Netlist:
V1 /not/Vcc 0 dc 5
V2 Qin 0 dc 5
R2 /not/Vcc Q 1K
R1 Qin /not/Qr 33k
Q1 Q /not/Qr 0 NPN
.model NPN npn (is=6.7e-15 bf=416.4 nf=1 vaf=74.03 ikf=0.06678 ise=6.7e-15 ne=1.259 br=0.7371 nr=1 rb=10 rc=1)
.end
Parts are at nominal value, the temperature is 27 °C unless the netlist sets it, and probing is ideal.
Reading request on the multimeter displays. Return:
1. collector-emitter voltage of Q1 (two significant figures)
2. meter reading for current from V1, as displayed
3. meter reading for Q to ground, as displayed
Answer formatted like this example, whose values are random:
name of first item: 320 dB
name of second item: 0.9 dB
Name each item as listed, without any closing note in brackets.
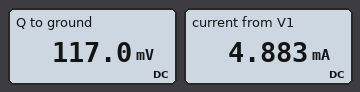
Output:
collector-emitter voltage of Q1: 120 mV
meter reading for current from V1, as displayed: 4.883 mA
meter reading for Q to ground, as displayed: 117.0 mV
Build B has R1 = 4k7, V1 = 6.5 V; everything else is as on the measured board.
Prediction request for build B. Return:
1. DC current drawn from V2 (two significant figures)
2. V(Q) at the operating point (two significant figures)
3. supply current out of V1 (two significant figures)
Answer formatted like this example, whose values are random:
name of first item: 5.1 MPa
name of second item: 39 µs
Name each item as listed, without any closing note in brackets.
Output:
DC current drawn from V2: 910 µA
V(Q) at the operating point: 75 mV
supply current out of V1: 6.4 mA
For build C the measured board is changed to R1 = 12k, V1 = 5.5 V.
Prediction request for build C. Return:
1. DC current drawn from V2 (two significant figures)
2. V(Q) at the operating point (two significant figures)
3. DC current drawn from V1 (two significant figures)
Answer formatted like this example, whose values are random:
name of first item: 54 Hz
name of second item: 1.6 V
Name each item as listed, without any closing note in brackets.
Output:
DC current drawn from V2: 360 µA
V(Q) at the operating point: 91 mV
DC current drawn from V1: 5.4 mA
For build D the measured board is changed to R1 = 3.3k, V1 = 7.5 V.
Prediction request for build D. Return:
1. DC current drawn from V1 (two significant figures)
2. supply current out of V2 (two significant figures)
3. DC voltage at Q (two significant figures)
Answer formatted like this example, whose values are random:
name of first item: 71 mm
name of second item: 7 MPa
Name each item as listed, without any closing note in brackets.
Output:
DC current drawn from V1: 7.4 mA
supply current out of V2: 1.3 mA
DC voltage at Q: 72 mV
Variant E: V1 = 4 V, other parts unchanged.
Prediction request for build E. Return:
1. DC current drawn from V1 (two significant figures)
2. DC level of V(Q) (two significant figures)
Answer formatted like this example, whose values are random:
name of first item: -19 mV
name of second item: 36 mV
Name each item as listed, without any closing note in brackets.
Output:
DC current drawn from V1: 3.9 mA
DC level of V(Q): 110 mV
